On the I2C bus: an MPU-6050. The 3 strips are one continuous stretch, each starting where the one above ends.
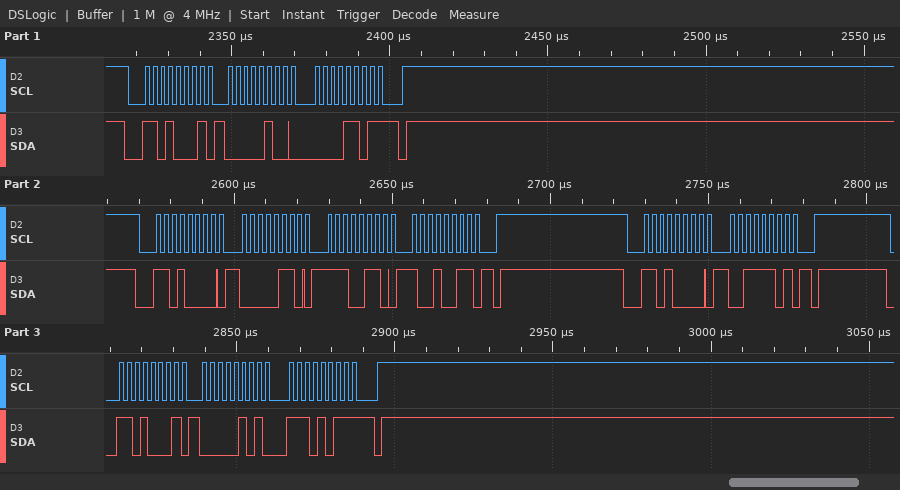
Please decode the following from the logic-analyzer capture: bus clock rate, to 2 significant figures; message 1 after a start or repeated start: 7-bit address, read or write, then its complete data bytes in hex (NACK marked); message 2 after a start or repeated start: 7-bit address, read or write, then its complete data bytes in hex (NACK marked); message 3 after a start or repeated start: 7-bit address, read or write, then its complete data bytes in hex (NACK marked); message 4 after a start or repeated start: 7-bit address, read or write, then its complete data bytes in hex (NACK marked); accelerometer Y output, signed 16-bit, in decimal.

400 kHz
0x68 read: 04 0D NACK
0x68 write: 06 E6 93
0x68 write: 3D
0x68 read: 05 EB NACK
1515
